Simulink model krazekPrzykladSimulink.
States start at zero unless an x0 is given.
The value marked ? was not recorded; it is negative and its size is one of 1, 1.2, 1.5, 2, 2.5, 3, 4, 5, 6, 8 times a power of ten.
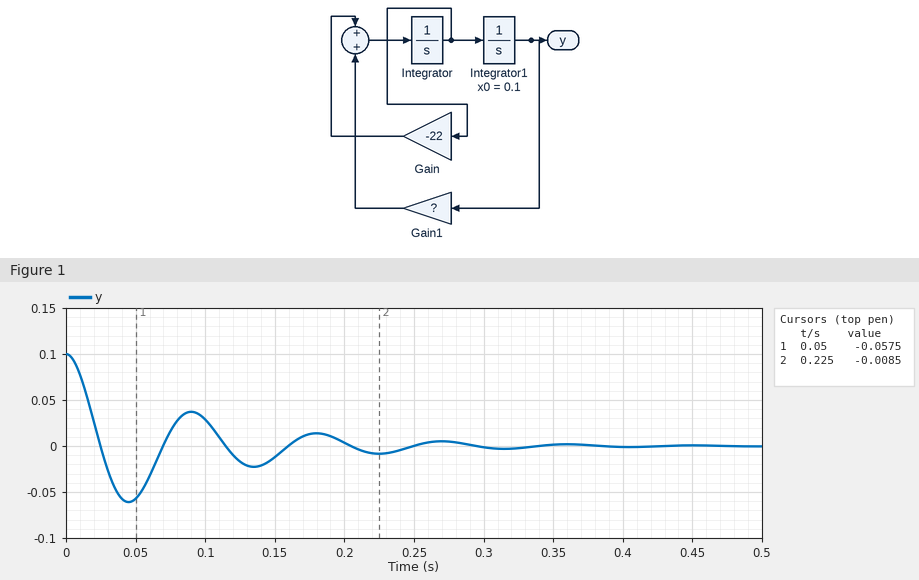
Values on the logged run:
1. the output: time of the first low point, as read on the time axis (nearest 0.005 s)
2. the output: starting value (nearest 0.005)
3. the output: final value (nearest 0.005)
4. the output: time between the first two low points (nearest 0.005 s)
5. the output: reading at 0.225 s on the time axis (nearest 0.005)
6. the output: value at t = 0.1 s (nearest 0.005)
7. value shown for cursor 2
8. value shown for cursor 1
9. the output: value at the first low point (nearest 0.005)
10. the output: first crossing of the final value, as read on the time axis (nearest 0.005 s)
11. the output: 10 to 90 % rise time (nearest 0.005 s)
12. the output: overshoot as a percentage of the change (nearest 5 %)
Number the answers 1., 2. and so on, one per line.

1. 0.045 s
2. 0.100
3. 0.000
4. 0.090 s
5. -0.010
6. 0.030
7. -0.0085
8. -0.0575
9. -0.060
10. 0.025 s
11. 0.015 s
12. 60 %
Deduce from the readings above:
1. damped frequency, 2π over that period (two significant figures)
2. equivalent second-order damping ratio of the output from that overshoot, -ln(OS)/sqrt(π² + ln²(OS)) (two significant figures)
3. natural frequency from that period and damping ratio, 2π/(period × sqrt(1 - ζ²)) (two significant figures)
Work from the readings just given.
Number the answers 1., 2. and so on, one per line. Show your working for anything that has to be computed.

1. 2π / 0.09 = 70 rad/s
2. ln(0.6) = -0.511; 0.511 / sqrt(9.870 + 0.261) = 0.16
3. 2π / (0.09 × sqrt(1 - 0.16²)) = 71 rad/s
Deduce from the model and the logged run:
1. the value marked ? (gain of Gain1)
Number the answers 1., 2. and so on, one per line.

1. -5000
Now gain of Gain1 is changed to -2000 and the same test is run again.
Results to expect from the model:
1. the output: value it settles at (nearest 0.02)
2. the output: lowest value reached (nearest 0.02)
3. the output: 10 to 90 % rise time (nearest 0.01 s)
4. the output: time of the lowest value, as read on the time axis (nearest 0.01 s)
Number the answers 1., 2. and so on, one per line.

1. 0.00
2. -0.04
3. 0.03 s
4. 0.07 s
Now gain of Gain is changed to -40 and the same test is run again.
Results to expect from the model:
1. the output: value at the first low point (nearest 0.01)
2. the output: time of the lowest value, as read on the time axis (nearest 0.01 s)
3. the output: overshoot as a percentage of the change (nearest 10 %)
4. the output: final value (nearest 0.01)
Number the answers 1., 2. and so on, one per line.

1. -0.04
2. 0.05 s
3. 40 %
4. 0.00
